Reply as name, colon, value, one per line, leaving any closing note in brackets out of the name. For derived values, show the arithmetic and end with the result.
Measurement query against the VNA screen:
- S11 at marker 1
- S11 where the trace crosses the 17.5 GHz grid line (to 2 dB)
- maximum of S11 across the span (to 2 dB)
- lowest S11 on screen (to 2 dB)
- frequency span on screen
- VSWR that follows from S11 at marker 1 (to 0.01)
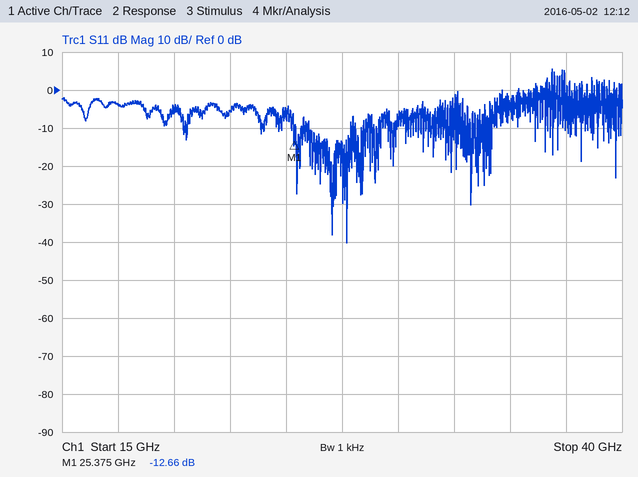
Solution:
S11 at marker 1: -12.66 dB
S11 where the trace crosses the 17.5 GHz grid line: -4 dB
maximum of S11 across the span: 6 dB
lowest S11 on screen: -40 dB
frequency span on screen: 25 GHz
VSWR that follows from S11 at marker 1: (1 + 0.2328)/(1 − 0.2328) ≈ 1.61
